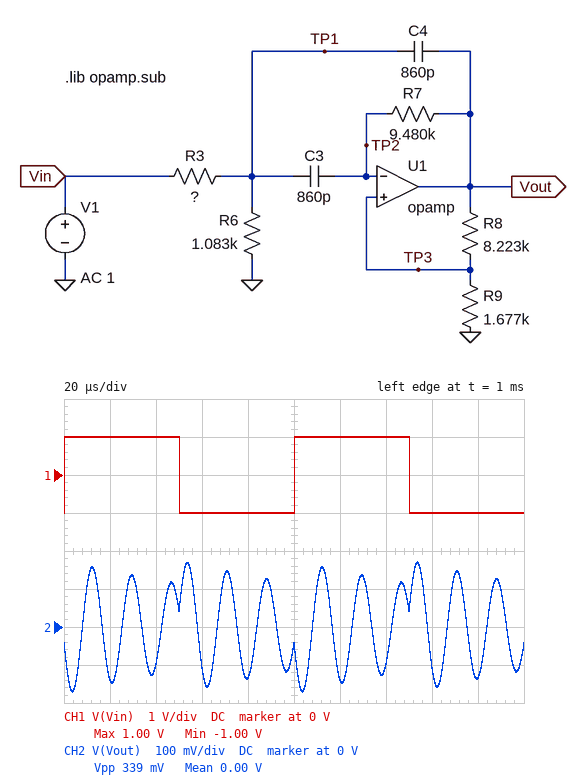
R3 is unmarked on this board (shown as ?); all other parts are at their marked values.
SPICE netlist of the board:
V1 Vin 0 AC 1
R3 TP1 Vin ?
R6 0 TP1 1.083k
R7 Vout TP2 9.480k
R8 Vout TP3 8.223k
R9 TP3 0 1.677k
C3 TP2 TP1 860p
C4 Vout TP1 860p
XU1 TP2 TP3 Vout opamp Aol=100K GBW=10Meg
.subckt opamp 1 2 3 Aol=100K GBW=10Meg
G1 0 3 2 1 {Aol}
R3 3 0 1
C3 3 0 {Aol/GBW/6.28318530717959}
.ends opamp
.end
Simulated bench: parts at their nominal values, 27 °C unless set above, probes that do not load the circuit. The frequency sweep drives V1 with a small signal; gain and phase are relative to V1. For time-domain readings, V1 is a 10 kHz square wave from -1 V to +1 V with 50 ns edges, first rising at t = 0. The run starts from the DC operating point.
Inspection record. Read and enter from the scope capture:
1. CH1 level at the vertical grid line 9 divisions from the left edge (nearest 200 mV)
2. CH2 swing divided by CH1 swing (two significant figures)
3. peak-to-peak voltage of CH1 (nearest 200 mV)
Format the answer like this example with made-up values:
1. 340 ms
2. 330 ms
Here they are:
1. -1.0 V
2. 0.17
3. 2.0 V
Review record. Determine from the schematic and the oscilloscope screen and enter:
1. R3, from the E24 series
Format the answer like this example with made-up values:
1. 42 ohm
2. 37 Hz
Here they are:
1. 27 kΩ
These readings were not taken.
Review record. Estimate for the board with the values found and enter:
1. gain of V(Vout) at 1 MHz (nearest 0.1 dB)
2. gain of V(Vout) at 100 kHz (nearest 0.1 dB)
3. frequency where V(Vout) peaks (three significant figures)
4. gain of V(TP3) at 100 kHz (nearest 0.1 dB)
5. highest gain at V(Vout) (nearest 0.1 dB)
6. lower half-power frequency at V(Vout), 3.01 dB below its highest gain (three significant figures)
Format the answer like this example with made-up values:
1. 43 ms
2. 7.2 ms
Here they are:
1. -41.9 dB
2. -18.3 dB
3. 58.2 kHz
4. -33.7 dB
5. 9.4 dB
6. 56.8 kHz
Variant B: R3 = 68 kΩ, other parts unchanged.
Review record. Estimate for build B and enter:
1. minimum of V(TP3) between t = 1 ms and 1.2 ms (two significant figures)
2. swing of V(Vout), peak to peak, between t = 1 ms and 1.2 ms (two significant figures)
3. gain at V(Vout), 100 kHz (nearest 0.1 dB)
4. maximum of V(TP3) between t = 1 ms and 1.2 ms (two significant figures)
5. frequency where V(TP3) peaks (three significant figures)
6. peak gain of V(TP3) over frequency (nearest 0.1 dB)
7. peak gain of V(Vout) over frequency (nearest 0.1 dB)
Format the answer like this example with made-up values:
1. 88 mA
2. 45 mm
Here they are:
1. -12 mV
2. 150 mV
3. -26.4 dB
4. 12 mV
5. 57.5 kHz
6. -16.4 dB
7. -0.9 dB
